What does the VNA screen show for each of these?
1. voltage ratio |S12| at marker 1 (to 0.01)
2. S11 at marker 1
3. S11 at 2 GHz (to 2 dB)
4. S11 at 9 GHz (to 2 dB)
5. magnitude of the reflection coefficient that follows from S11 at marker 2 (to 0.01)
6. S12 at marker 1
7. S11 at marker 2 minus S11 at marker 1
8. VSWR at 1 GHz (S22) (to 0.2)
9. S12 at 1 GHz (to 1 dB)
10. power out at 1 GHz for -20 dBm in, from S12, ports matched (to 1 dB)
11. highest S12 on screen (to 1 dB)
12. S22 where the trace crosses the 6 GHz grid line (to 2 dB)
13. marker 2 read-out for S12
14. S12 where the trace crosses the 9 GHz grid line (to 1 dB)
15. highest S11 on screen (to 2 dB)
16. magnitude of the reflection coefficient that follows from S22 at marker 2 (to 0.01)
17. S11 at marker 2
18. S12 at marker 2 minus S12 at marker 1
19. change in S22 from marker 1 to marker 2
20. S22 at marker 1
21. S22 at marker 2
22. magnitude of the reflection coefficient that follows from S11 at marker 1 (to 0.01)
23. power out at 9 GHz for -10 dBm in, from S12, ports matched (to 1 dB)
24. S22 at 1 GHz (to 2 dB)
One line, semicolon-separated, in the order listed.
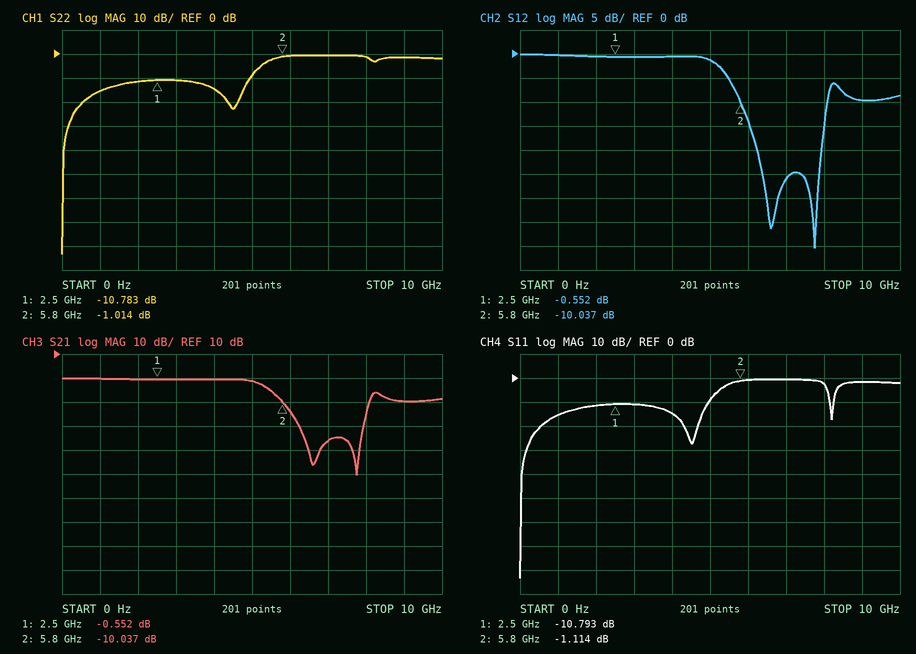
0.94; -10.793 dB; -12 dB; -2 dB; 0.88; -0.552 dB; 9.679 dB; 1.4; 0 dB; -20 dBm; 0 dB; 0 dB; -10.037 dB; -10 dB; 0 dB; 0.89; -1.114 dB; -9.485 dB; 9.769 dB; -10.783 dB; -1.014 dB; 0.29; -20 dBm; -16 dB
